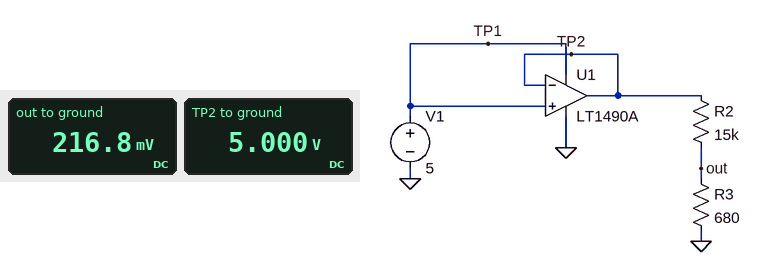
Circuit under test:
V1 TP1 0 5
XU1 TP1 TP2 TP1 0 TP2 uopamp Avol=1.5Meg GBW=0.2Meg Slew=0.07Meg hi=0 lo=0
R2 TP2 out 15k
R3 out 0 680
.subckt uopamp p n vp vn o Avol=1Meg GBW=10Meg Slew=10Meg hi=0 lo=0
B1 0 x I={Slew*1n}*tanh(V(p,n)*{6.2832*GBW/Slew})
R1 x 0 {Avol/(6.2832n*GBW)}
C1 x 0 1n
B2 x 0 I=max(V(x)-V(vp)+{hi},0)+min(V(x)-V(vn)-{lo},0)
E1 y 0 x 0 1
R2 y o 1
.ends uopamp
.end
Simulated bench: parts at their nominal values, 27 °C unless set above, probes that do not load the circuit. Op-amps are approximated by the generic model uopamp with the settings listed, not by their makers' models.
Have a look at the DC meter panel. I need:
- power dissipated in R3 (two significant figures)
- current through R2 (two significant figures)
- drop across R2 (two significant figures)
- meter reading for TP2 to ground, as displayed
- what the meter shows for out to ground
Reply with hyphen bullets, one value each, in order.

- 69 µW
- 320 µA
- 4.8 V
- 5.000 V
- 216.8 mV
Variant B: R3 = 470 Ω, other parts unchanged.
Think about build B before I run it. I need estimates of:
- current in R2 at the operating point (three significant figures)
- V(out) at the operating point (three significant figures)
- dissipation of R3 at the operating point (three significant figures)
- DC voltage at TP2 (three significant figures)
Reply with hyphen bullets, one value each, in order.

- 323 µA
- 152 mV
- 49.1 µW
- 5.00 V
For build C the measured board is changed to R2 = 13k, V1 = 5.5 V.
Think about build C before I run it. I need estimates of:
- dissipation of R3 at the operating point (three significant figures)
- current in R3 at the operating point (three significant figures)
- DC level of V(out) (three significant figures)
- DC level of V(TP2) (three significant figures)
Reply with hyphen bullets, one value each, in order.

- 110 µW
- 402 µA
- 273 mV
- 5.50 V
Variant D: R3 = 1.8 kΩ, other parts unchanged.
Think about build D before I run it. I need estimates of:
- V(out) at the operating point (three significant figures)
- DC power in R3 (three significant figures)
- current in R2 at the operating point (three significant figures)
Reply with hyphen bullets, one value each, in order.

- 536 mV
- 159 µW
- 298 µA
